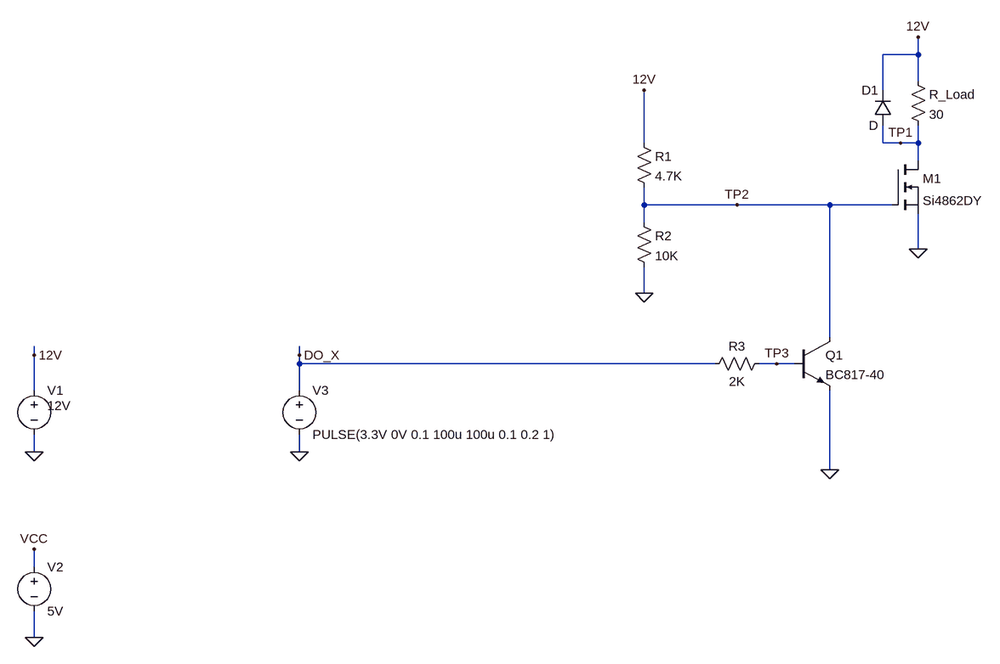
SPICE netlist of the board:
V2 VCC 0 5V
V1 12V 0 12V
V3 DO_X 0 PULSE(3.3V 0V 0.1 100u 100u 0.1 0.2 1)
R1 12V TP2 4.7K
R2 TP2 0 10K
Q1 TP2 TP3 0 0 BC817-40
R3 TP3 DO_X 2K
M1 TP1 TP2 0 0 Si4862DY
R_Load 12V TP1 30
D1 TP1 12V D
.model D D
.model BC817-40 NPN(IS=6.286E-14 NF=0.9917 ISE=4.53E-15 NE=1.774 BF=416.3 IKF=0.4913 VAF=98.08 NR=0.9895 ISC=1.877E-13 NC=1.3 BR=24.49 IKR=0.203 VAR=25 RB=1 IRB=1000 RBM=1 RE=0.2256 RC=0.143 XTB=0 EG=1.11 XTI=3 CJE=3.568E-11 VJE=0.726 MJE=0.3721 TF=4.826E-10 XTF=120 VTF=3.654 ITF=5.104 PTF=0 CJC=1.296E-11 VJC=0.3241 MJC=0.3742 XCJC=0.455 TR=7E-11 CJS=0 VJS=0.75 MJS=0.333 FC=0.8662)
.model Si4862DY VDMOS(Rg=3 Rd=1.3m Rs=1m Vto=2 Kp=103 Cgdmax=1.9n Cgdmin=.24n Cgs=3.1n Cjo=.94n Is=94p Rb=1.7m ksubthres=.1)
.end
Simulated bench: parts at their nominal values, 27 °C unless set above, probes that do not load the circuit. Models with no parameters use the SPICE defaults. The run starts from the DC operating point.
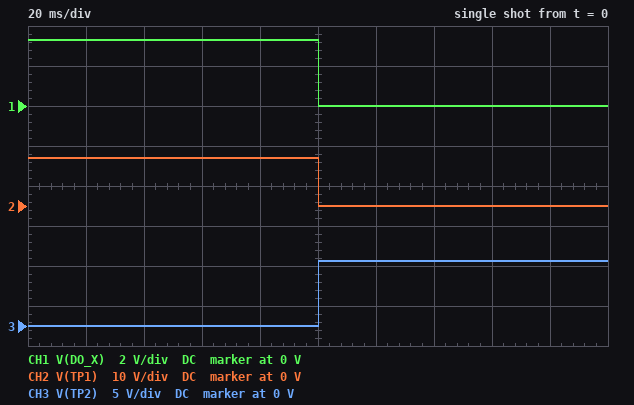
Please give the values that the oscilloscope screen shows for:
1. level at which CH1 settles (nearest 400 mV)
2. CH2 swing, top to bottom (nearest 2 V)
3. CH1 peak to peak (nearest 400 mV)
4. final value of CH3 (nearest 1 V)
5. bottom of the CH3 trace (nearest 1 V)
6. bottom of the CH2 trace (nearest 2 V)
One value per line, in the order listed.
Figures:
0 V
12 V
3.2 V
8 V
0 V
0 V
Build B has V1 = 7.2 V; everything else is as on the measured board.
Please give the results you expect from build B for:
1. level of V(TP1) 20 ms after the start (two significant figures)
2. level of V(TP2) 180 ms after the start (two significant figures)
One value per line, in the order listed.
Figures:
7.2 V
4.9 V
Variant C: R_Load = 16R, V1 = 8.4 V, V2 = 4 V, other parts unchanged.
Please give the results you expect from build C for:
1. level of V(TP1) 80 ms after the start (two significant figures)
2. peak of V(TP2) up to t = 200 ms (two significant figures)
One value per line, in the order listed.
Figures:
8.4 V
5.7 V
